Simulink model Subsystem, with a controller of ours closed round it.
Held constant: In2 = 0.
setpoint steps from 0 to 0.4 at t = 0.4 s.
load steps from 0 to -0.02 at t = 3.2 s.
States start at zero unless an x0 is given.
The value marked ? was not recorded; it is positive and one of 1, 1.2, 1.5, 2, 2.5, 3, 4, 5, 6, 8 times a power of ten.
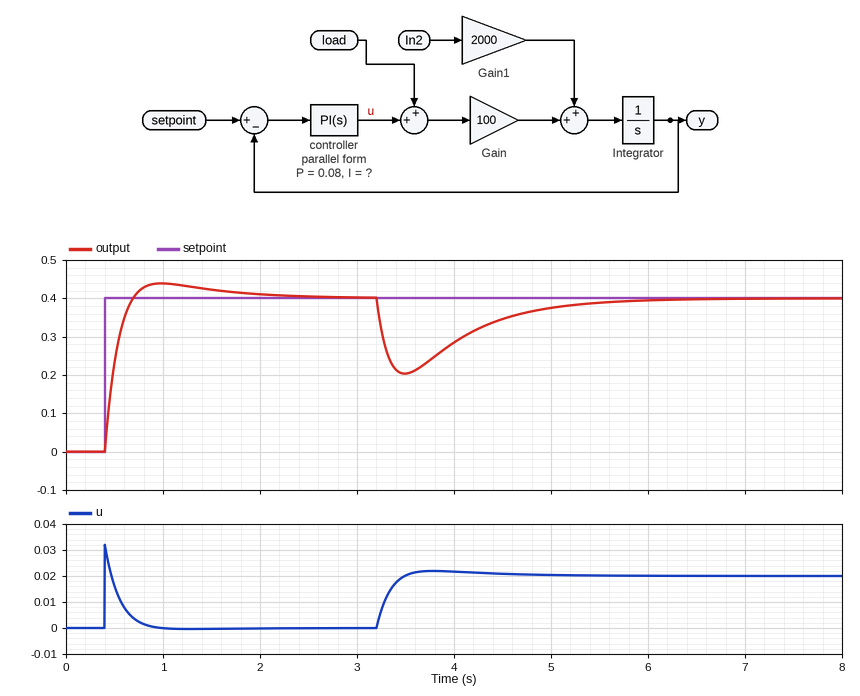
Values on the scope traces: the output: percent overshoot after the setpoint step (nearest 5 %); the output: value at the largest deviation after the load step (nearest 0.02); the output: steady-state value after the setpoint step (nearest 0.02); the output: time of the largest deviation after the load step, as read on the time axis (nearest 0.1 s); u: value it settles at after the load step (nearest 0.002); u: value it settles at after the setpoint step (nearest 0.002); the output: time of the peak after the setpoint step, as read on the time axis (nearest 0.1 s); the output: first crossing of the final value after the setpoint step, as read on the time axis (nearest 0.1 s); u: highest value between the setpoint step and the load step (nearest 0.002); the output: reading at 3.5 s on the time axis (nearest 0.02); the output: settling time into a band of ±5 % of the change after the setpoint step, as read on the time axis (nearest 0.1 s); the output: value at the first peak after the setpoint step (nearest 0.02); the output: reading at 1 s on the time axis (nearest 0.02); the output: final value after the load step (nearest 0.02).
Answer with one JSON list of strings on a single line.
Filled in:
["10 %", "0.20", "0.40", "3.5 s", "0.020", "0.000", "1.0 s", "0.7 s", "0.032", "0.20", "1.6 s", "0.44", "0.44", "0.40"]
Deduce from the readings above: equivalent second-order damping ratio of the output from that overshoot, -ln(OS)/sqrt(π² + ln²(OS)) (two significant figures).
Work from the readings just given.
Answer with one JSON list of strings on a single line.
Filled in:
["0.59"]
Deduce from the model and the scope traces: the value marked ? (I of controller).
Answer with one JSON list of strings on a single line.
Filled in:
["0.1"]
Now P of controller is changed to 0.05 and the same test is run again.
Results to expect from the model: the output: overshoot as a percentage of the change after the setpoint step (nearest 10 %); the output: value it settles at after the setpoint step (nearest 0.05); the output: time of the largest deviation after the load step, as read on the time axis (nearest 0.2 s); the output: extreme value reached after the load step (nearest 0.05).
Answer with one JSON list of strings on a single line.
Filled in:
["20 %", "0.40", "3.6 s", "0.15"]
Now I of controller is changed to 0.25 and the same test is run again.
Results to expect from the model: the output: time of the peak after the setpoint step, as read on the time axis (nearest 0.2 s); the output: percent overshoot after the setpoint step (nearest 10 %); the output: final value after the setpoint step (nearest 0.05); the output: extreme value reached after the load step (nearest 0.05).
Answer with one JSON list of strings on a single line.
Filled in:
["0.8 s", "20 %", "0.40", "0.25"]
